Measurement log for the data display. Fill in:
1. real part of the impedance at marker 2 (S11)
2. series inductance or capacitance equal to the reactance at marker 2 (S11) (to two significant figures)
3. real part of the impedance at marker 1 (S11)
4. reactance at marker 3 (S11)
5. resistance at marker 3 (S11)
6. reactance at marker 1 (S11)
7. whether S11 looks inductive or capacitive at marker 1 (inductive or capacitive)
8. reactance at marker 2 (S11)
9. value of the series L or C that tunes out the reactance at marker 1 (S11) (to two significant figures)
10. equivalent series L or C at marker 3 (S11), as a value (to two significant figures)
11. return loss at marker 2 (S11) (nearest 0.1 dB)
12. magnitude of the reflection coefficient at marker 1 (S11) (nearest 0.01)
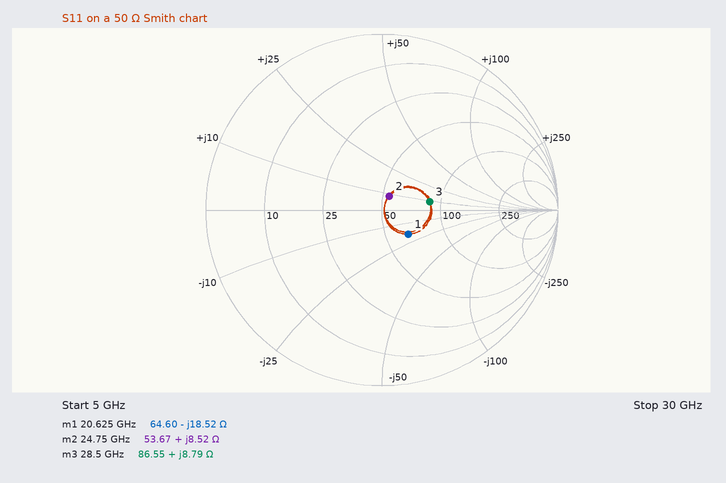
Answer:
53.67 Ω
55 pH
64.60 Ω
+8.79 Ω
86.55 Ω
-18.52 Ω
capacitive
+8.52 Ω
140 pH
49 pH
21.0 dB
0.20
